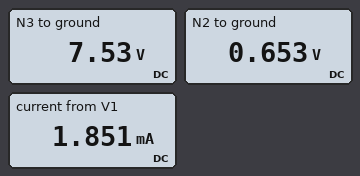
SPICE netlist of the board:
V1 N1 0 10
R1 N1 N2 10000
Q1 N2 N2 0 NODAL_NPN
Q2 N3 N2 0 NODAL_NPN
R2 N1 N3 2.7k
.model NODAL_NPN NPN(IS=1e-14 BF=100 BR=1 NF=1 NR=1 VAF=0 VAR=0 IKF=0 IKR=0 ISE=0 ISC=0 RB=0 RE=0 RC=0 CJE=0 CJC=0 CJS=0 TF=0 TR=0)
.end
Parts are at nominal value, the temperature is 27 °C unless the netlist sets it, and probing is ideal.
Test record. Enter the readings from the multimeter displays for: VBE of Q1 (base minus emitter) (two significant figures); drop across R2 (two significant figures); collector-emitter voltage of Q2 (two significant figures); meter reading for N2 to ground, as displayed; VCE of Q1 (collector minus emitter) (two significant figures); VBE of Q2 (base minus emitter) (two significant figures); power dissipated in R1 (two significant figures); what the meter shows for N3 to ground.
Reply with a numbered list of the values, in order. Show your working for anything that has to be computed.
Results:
1. 653 mV = 650 mV
2. 10 V - 7.53 V = 2.5 V
3. 7.53 V = 7.5 V
4. 0.653 V
5. 653 mV = 650 mV
6. 653 mV = 650 mV
7. (10 V - 653 mV)^2 / 10 kΩ = 8.7 mW
8. 7.53 V
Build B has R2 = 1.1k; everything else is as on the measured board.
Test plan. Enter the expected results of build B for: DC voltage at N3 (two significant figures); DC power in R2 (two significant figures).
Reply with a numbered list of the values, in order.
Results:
1. 9.0 V
2. 920 µW
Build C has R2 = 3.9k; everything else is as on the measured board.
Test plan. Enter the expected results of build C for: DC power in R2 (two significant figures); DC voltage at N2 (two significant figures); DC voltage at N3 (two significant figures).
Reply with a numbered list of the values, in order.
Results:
1. 3.3 mW
2. 650 mV
3. 6.4 V
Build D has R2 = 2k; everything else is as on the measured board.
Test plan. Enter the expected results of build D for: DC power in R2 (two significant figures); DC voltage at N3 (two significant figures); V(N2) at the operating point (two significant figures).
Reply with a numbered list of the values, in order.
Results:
1. 1.7 mW
2. 8.2 V
3. 650 mV
